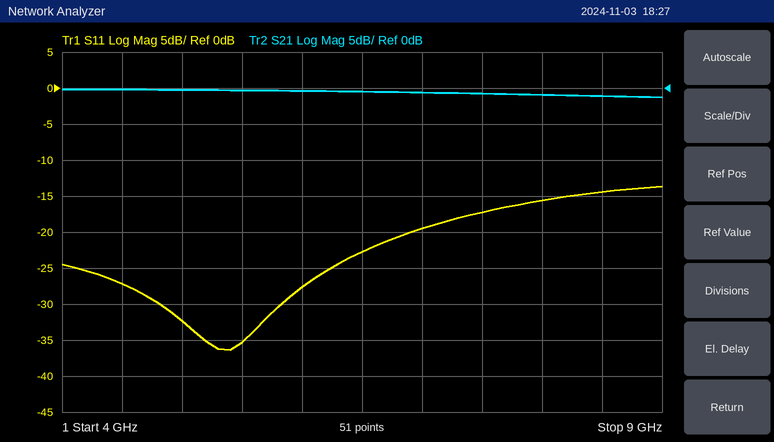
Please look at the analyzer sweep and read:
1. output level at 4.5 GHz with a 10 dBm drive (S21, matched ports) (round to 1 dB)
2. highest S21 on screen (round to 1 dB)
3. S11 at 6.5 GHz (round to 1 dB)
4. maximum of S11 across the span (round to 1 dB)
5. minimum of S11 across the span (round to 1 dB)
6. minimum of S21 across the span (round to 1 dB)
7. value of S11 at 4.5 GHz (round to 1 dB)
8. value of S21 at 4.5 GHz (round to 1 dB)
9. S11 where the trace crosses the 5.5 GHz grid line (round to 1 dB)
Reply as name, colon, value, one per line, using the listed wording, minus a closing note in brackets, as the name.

output level at 4.5 GHz with a 10 dBm drive (S21, matched ports): 10 dBm
highest S21 on screen: 0 dB
S11 at 6.5 GHz: -23 dB
maximum of S11 across the span: -14 dB
minimum of S11 across the span: -36 dB
minimum of S21 across the span: -1 dB
value of S11 at 4.5 GHz: -27 dB
value of S21 at 4.5 GHz: 0 dB
S11 where the trace crosses the 5.5 GHz grid line: -35 dB
